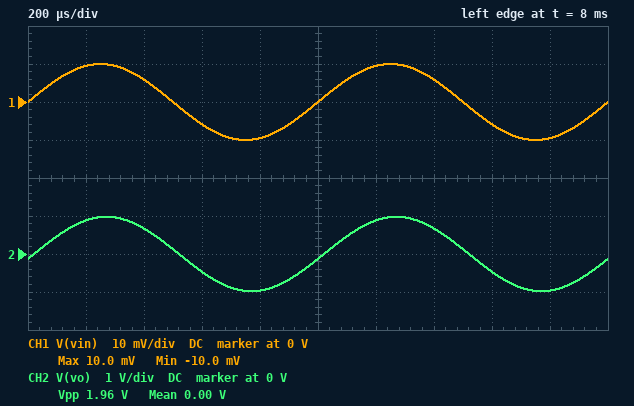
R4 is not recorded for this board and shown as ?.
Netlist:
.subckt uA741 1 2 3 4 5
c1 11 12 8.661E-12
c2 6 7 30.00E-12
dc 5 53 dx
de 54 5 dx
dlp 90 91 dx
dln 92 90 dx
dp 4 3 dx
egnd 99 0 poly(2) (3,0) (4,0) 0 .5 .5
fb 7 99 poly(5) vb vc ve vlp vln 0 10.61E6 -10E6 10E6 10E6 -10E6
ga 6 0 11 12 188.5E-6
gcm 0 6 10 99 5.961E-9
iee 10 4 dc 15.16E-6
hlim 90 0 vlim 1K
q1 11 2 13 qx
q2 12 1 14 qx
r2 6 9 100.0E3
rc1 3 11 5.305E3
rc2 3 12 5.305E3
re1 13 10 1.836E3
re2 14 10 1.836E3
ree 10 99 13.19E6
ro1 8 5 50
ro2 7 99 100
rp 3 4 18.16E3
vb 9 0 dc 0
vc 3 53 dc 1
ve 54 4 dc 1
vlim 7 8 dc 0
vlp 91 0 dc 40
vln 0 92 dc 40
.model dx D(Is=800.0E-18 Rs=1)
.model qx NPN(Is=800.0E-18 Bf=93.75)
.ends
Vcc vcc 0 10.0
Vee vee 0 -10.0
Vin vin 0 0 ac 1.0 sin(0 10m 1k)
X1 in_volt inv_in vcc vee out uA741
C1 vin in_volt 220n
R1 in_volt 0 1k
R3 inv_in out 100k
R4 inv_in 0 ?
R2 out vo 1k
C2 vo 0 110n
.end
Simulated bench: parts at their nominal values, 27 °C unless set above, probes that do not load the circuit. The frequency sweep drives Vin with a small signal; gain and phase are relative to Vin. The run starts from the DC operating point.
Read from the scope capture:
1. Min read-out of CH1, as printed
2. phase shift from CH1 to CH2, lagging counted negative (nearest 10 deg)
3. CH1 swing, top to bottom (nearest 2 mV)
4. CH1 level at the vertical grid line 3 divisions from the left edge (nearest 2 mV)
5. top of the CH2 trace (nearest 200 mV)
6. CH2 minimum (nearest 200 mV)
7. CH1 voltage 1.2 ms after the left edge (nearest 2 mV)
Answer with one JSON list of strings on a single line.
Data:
["-10.0 mV", "-10 deg", "20 mV", "-6 mV", "1.0 V", "-1.0 V", "10 mV"]
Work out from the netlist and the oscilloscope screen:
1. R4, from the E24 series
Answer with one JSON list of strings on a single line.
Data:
["680 Ω"]
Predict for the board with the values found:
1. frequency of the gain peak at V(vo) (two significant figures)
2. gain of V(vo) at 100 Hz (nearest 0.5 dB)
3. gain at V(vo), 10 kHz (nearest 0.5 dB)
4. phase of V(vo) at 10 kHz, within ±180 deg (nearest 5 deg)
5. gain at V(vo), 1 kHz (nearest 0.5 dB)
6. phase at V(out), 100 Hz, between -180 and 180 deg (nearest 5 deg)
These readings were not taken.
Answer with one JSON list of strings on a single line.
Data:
["1.0 kHz", "26.0 dB", "21.0 dB", "-135 deg", "40.0 dB", "80 deg"]
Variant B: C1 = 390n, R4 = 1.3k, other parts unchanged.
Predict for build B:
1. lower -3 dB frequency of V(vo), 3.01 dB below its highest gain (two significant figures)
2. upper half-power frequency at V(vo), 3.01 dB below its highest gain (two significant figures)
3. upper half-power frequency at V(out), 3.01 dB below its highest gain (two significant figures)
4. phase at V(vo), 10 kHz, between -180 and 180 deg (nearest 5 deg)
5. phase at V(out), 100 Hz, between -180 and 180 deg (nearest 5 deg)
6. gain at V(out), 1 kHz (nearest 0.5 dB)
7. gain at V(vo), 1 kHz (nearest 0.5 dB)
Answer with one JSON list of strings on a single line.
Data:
["280 Hz", "2.1 kHz", "13 kHz", "-120 deg", "75 deg", "37.0 dB", "35.5 dB"]
